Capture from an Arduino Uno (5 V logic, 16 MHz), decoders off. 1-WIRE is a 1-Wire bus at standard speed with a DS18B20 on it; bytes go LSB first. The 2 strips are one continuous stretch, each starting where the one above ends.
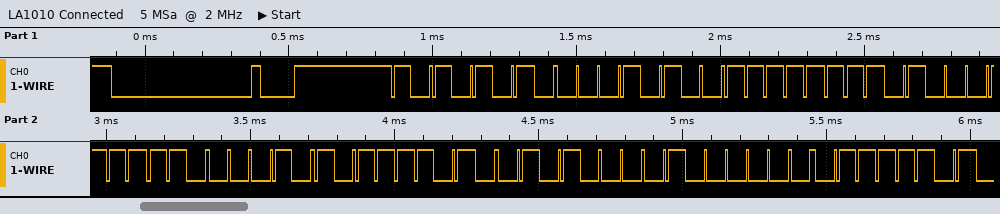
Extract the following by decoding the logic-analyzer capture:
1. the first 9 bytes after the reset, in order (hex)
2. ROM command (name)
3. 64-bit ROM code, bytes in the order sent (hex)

55 28 FF E2 43 BD 14 02 BE
Match ROM
28 FF E2 43 BD 14 02 BE
